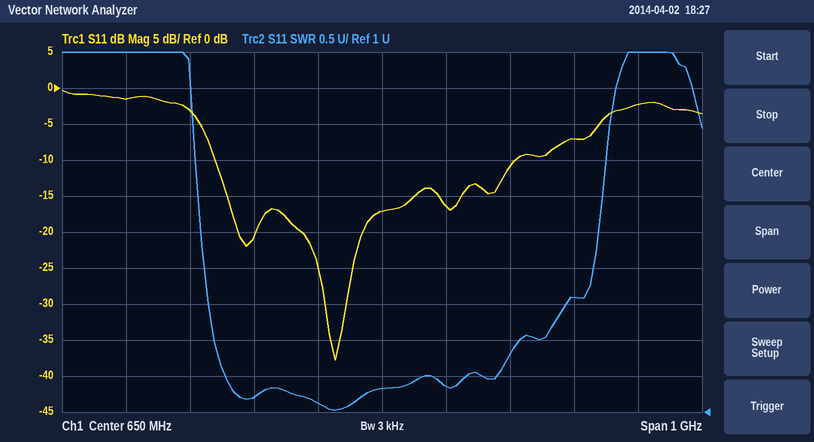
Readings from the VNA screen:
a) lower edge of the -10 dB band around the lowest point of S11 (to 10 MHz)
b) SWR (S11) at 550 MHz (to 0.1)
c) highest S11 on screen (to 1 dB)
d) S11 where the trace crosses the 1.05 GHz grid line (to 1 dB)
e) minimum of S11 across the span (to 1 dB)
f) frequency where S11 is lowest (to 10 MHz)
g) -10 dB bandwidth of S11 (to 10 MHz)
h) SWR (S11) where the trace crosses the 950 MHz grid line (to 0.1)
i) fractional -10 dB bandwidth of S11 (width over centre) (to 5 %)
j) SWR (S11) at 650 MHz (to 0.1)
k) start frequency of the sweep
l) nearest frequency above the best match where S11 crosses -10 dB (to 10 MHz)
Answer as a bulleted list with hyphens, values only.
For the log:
- 390 MHz
- 1.1
- 0 dB
- -2 dB
- -38 dB
- 580 MHz
- 470 MHz
- 2.6
- 75 %
- 1.3
- 150 MHz
- 860 MHz
